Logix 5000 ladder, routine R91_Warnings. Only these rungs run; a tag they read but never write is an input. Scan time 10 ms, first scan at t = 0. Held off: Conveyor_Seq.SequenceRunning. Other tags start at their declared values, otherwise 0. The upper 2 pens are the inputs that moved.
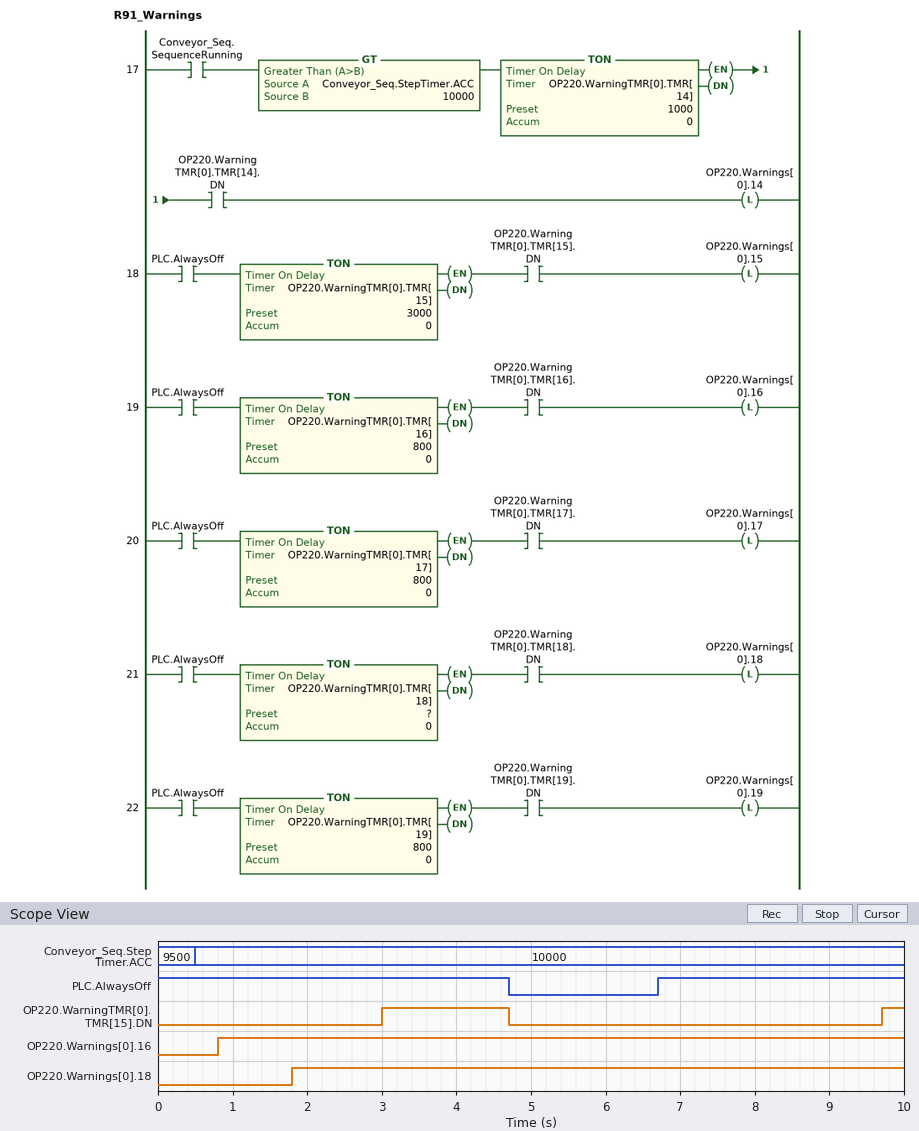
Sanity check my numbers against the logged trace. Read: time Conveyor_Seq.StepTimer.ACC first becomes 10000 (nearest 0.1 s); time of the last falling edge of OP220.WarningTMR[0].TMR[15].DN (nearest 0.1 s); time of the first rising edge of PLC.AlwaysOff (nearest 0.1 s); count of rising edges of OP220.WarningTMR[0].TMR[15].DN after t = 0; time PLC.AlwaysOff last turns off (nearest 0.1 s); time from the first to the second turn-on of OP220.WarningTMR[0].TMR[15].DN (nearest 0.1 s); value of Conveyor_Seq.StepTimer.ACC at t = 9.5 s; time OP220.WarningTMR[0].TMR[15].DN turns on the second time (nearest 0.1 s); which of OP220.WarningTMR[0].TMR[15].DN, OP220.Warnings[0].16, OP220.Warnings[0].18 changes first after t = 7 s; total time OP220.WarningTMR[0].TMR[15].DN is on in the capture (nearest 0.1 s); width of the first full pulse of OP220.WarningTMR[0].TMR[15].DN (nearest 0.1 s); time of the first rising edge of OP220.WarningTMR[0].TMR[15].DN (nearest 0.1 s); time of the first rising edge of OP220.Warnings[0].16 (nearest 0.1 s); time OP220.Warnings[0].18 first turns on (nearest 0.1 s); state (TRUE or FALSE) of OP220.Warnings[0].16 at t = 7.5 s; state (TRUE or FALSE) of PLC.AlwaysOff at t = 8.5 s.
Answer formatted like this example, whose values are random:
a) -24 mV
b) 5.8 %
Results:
a) 0.5 s
b) 4.7 s
c) 6.7 s
d) 2
e) 4.7 s
f) 6.7 s
g) 10000
h) 9.7 s
i) OP220.WarningTMR[0].TMR[15].DN
j) 2.0 s
k) 1.7 s
l) 3.0 s
m) 0.8 s
n) 1.8 s
o) TRUE
p) TRUE
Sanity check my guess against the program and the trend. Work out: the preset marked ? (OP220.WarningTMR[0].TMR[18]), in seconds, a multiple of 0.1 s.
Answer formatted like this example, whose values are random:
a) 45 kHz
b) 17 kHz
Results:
a) 1.8 s
